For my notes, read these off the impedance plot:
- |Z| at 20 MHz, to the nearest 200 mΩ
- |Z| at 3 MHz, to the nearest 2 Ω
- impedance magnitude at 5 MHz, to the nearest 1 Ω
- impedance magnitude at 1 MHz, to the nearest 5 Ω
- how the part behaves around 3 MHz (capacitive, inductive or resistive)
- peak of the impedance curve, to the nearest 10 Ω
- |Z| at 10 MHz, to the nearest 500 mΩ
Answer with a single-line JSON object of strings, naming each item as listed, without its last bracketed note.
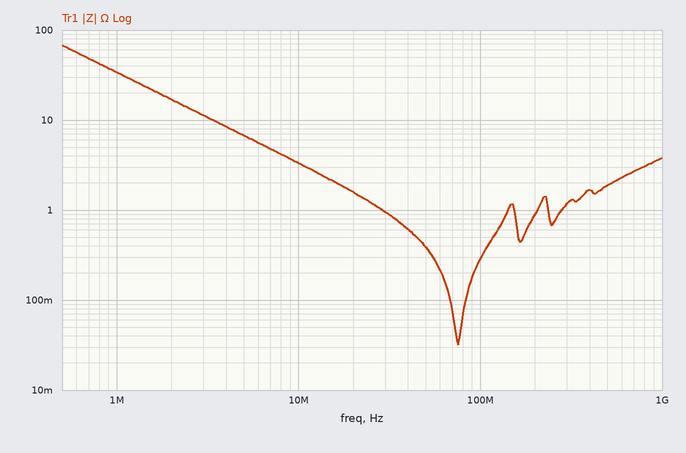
{"|Z| at 20 MHz, to the nearest 200 mΩ": "1.6 Ω", "|Z| at 3 MHz, to the nearest 2 Ω": "12 Ω", "impedance magnitude at 5 MHz, to the nearest 1 Ω": "7 Ω", "impedance magnitude at 1 MHz, to the nearest 5 Ω": "35 Ω", "how the part behaves around 3 MHz": "capacitive", "peak of the impedance curve, to the nearest 10 Ω": "70 Ω", "|Z| at 10 MHz, to the nearest 500 mΩ": "3.5 Ω"}
